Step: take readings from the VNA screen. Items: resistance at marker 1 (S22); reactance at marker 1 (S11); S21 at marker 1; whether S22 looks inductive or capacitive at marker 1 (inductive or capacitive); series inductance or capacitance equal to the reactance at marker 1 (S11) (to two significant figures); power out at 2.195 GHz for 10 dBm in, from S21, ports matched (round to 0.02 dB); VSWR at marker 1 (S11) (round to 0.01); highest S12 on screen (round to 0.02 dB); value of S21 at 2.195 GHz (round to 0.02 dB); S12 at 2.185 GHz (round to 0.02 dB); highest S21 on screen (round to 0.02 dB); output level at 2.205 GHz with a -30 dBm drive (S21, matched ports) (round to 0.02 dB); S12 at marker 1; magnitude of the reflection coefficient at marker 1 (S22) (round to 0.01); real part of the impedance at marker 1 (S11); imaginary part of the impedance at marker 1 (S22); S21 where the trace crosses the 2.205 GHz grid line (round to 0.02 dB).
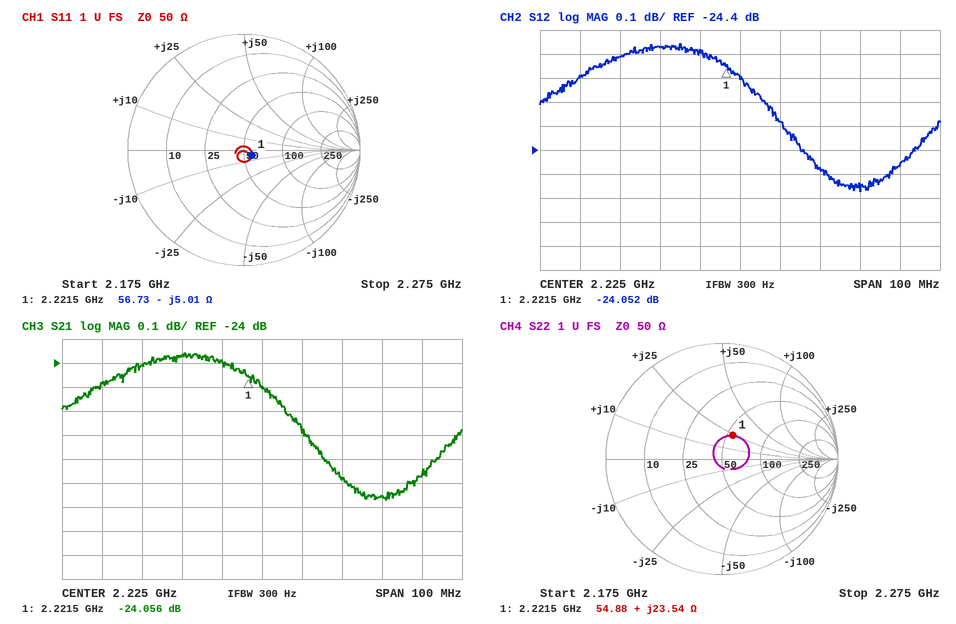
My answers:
54.88 Ω
-5.01 Ω
-24.056 dB
inductive
14 pF
-14.00 dBm
1.17
-23.96 dB
-24.00 dB
-24.10 dB
-23.96 dB
-53.96 dBm
-24.052 dB
0.22
56.73 Ω
+23.54 Ω
-23.96 dB
